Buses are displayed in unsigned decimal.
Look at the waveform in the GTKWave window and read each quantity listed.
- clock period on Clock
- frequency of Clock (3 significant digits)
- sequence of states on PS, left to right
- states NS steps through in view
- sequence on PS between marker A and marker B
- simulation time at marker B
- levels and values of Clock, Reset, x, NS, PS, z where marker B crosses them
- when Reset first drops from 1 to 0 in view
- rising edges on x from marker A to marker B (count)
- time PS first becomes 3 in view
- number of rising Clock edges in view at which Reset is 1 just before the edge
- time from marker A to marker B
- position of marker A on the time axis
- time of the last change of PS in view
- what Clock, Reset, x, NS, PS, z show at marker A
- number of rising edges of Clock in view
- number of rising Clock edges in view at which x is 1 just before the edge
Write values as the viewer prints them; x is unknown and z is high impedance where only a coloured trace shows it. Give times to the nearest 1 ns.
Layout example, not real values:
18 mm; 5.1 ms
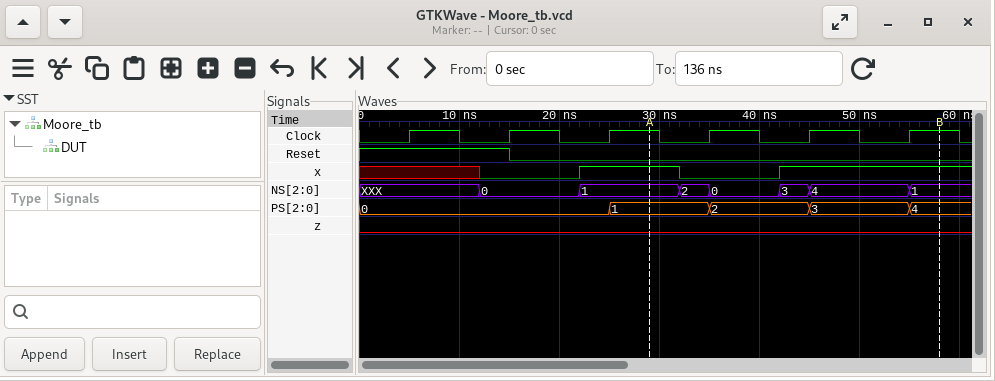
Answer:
10 ns; 100 MHz; 0, 1, 2, 3, 4; XXX, 0, 1, 2, 0, 3, 4, 1; 1, 2, 3, 4; 58 ns; Clock=1, Reset=0, x=1, NS=1, PS=4, z=0; 15 ns; 1; 45 ns; 2; 29 ns; 29 ns; 55 ns; Clock=1, Reset=0, x=1, NS=1, PS=1, z=0; 6; 3
